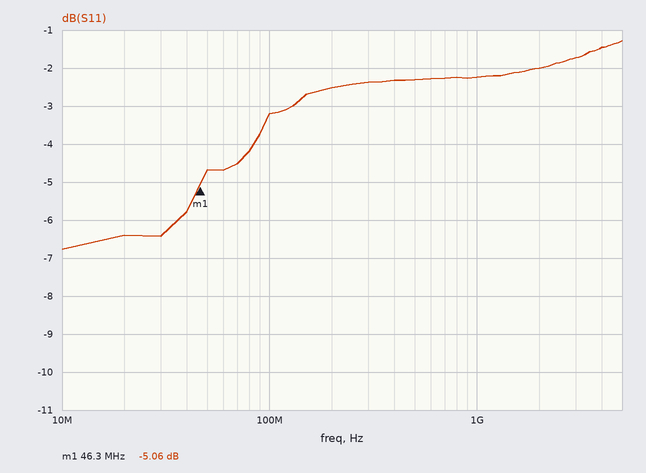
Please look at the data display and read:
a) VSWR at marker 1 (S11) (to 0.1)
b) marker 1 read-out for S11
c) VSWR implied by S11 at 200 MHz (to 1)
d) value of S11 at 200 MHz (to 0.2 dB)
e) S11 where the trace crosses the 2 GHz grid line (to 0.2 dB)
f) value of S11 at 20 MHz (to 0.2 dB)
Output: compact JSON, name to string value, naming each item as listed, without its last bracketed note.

{"VSWR at marker 1 (S11)": "3.5", "marker 1 read-out for S11": "-5.06 dB", "VSWR implied by S11 at 200 MHz": "7", "value of S11 at 200 MHz": "-2.6 dB", "S11 where the trace crosses the 2 GHz grid line": "-2.0 dB", "value of S11 at 20 MHz": "-6.4 dB"}
